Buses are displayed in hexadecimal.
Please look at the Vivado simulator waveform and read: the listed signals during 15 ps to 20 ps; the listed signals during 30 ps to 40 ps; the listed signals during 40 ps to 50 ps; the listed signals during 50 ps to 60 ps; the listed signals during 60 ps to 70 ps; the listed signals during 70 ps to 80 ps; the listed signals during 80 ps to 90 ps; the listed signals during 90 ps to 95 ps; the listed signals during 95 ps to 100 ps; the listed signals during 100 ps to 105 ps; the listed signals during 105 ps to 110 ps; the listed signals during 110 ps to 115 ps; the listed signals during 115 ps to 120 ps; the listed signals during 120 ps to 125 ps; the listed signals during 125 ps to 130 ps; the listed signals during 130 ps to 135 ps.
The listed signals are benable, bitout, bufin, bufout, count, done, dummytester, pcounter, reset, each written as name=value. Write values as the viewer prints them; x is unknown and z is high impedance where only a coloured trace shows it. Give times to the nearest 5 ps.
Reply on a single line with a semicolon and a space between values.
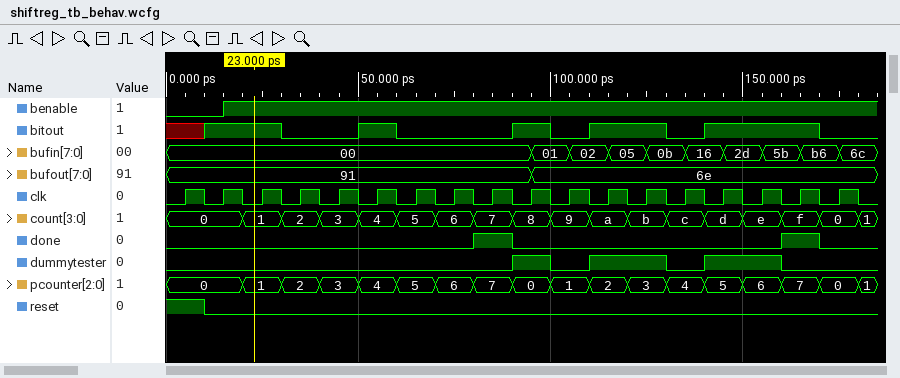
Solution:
benable=1, bitout=1, bufin=00, bufout=91, count=0, done=0, dummytester=0, pcounter=0, reset=0; benable=1, bitout=0, bufin=00, bufout=91, count=2, done=0, dummytester=0, pcounter=2, reset=0; benable=1, bitout=0, bufin=00, bufout=91, count=3, done=0, dummytester=0, pcounter=3, reset=0; benable=1, bitout=1, bufin=00, bufout=91, count=4, done=0, dummytester=0, pcounter=4, reset=0; benable=1, bitout=0, bufin=00, bufout=91, count=5, done=0, dummytester=0, pcounter=5, reset=0; benable=1, bitout=0, bufin=00, bufout=91, count=6, done=0, dummytester=0, pcounter=6, reset=0; benable=1, bitout=0, bufin=00, bufout=91, count=7, done=1, dummytester=0, pcounter=7, reset=0; benable=1, bitout=1, bufin=00, bufout=91, count=8, done=0, dummytester=1, pcounter=0, reset=0; benable=1, bitout=1, bufin=01, bufout=6e, count=8, done=0, dummytester=1, pcounter=0, reset=0; benable=1, bitout=0, bufin=01, bufout=6e, count=9, done=0, dummytester=0, pcounter=1, reset=0; benable=1, bitout=0, bufin=02, bufout=6e, count=9, done=0, dummytester=0, pcounter=1, reset=0; benable=1, bitout=1, bufin=02, bufout=6e, count=a, done=0, dummytester=1, pcounter=2, reset=0; benable=1, bitout=1, bufin=05, bufout=6e, count=a, done=0, dummytester=1, pcounter=2, reset=0; benable=1, bitout=1, bufin=05, bufout=6e, count=b, done=0, dummytester=1, pcounter=3, reset=0; benable=1, bitout=1, bufin=0b, bufout=6e, count=b, done=0, dummytester=1, pcounter=3, reset=0; benable=1, bitout=0, bufin=0b, bufout=6e, count=c, done=0, dummytester=0, pcounter=4, reset=0
